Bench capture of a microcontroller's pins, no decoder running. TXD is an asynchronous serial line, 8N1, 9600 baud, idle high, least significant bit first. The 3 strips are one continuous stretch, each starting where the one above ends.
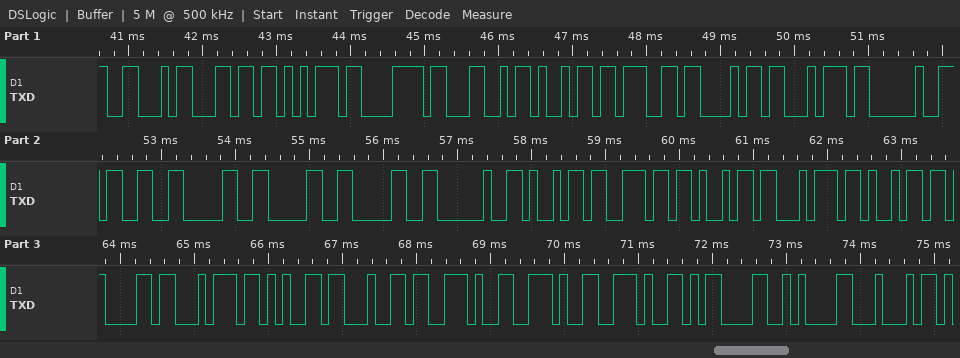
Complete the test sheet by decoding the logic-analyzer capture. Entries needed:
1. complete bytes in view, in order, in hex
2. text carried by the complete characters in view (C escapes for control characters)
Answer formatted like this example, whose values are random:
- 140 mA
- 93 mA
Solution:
- 46 6C 75 78 4C 69 67 68 74 20 33 30 30 30 20 69 6E 69 74 69 61 74 65 64 2E 2E 2E 0D 0A 44
- "FluxLight 3000 initiated...\r\nD"
